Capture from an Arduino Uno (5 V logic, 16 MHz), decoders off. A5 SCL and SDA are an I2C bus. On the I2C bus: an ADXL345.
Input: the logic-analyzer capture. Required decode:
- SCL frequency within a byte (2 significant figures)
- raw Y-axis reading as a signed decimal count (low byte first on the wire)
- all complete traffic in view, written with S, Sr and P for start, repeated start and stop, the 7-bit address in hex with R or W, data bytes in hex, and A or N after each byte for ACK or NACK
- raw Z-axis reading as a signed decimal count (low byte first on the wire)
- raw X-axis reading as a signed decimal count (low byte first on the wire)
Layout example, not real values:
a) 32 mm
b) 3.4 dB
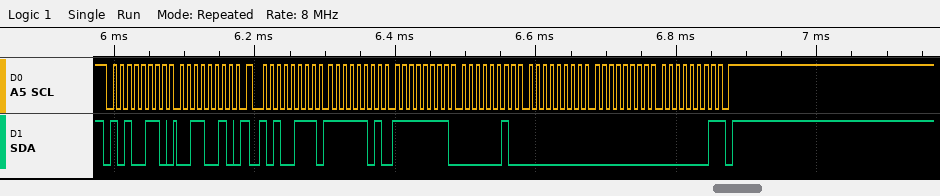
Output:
a) 100 kHz
b) 2
c) S 53W A 32 A Sr 53R A FD A FF A 02 A 00 A 00 A 01 N P
d) 256
e) -3
